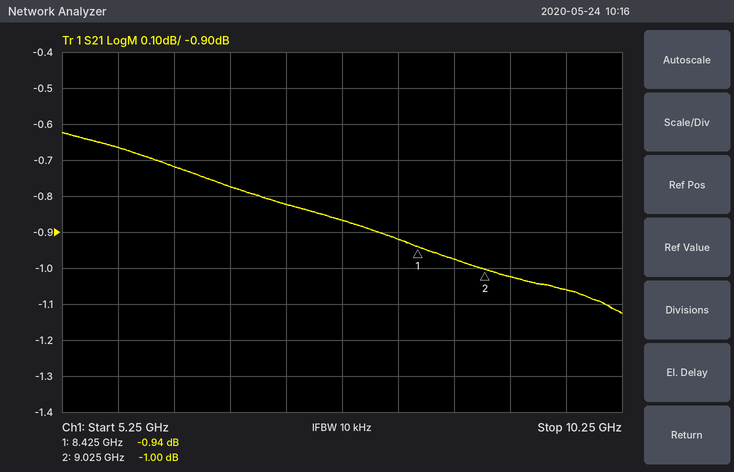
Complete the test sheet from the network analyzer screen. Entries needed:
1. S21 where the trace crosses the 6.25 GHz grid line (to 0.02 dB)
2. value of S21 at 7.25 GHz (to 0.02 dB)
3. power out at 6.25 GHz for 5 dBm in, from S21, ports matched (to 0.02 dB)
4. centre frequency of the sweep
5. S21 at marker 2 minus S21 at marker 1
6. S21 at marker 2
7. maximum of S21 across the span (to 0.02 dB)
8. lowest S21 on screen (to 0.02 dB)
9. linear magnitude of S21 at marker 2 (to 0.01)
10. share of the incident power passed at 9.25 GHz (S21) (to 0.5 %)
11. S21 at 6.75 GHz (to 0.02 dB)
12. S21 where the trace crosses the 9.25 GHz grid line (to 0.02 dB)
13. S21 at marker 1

-0.72 dB
-0.82 dB
4.28 dBm
7.75 GHz
-0.06 dB
-1.00 dB
-0.62 dB
-1.12 dB
0.89
79.0 %
-0.78 dB
-1.02 dB
-0.94 dB
